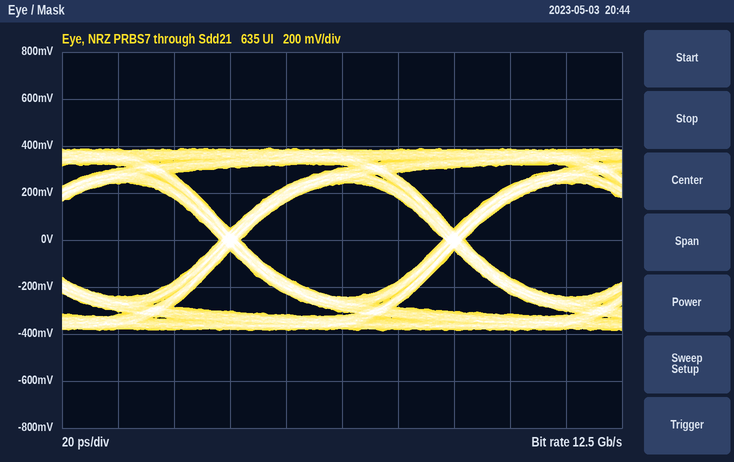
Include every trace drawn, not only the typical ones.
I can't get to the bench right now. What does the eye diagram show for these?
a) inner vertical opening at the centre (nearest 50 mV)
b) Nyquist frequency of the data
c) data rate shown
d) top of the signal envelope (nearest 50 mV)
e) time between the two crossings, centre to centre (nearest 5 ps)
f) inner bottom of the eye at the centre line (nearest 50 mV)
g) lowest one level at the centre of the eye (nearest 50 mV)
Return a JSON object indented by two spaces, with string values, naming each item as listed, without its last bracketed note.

{
  "inner vertical opening at the centre": "500 mV",
  "Nyquist frequency of the data": "6.25 GHz",
  "data rate shown": "12.5 Gb/s",
  "top of the signal envelope": "400 mV",
  "time between the two crossings, centre to centre": "80 ps",
  "inner bottom of the eye at the centre line": "-250 mV",
  "lowest one level at the centre of the eye": "250 mV"
}
